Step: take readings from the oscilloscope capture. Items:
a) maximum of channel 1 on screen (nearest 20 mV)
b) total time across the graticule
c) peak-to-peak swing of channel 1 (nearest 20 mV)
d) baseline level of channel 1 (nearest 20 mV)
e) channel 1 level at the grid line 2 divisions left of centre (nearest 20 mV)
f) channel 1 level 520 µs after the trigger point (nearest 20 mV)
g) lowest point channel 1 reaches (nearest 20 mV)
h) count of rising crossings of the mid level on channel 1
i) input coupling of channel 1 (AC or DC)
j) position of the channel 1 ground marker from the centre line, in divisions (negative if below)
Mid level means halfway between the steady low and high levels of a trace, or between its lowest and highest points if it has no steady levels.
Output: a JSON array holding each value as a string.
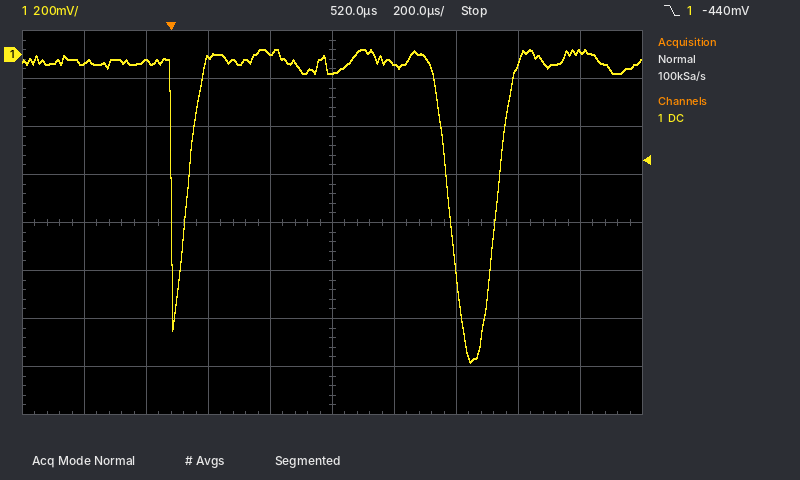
["20 mV", "2 ms", "1.30 V", "-40 mV", "-20 mV", "-80 mV", "-1.28 V", "2", "DC", "+3.5 div"]
